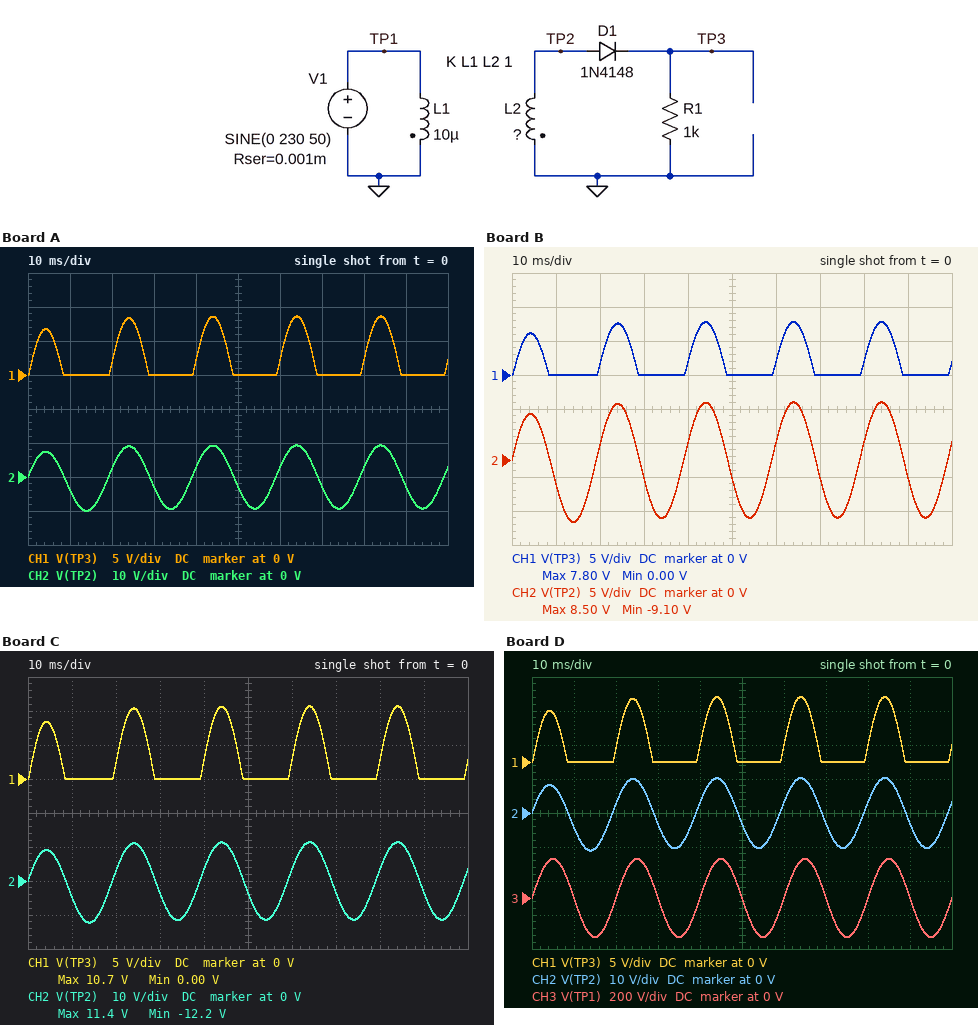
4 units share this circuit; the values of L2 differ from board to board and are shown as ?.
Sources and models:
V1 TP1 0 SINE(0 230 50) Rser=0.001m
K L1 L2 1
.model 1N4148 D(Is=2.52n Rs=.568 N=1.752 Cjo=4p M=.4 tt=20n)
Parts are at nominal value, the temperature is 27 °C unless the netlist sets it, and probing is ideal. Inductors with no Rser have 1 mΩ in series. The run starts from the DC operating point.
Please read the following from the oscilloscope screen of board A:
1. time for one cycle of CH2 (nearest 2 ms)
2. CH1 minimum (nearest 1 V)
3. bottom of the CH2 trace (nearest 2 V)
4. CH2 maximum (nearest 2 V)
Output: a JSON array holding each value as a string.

["20 ms", "0 V", "-10 V", "10 V"]
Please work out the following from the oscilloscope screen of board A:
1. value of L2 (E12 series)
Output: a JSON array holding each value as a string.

["18 nH"]
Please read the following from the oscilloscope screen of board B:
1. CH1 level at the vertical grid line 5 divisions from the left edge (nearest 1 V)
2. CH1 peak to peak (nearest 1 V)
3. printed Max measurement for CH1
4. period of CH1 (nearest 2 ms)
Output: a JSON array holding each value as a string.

["0 V", "8 V", "7.80 V", "20 ms"]
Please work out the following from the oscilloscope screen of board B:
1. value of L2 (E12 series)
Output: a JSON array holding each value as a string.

["15 nH"]
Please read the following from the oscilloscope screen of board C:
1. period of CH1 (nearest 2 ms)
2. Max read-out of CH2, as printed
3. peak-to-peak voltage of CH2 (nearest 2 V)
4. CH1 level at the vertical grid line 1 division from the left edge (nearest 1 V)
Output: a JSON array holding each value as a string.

["20 ms", "11.4 V", "24 V", "0 V"]
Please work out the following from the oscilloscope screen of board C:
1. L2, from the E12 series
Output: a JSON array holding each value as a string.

["27 nH"]
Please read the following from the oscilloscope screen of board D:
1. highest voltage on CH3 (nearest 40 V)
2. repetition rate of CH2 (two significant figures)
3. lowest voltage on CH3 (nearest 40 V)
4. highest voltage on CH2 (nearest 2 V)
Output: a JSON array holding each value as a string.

["240 V", "50 Hz", "-240 V", "10 V"]
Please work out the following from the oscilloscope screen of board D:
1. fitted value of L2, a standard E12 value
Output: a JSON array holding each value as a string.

["22 nH"]
